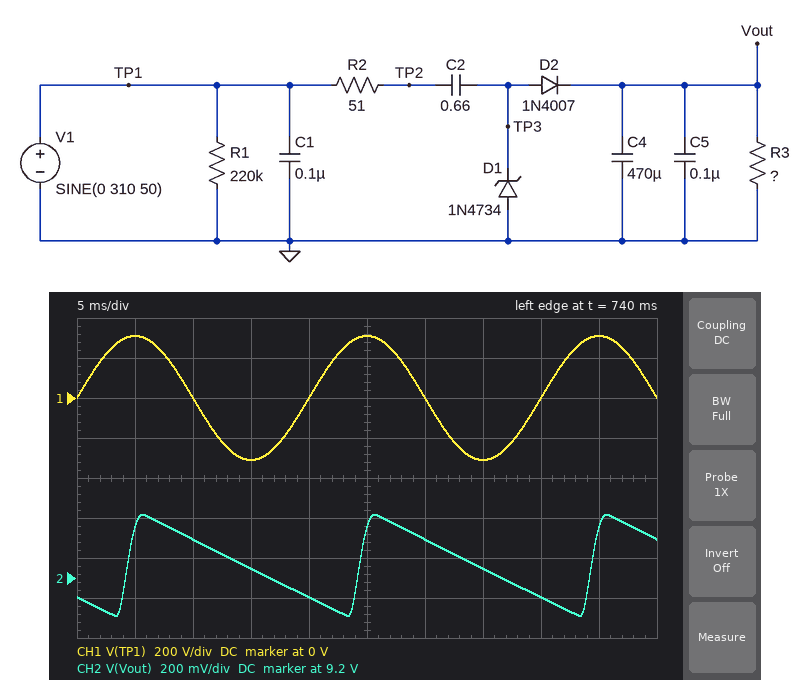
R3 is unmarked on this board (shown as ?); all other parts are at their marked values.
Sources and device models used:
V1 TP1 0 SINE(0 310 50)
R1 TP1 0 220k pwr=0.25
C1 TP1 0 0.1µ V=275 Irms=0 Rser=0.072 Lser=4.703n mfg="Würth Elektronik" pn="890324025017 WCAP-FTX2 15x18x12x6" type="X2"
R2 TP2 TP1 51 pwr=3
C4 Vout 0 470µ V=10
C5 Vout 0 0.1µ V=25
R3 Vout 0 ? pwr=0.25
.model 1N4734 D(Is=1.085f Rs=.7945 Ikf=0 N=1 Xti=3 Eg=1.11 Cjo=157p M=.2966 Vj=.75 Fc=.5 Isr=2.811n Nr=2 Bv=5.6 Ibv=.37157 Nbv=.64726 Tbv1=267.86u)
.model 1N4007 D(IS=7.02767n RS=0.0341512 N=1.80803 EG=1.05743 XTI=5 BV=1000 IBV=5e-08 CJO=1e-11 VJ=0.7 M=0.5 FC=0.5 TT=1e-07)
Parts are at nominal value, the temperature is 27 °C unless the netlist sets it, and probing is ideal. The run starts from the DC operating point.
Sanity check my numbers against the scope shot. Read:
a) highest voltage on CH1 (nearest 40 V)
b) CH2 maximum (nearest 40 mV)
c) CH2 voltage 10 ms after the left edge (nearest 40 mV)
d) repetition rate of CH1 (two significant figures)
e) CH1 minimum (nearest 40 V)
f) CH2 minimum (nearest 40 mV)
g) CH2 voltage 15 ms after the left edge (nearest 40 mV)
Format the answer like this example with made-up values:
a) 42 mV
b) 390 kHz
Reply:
a) 320 V
b) 9.52 V
c) 9.40 V
d) 50 Hz
e) -320 V
f) 9.00 V
g) 9.24 V
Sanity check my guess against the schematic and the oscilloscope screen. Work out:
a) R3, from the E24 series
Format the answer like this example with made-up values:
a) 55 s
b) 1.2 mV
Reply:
a) 680 Ω
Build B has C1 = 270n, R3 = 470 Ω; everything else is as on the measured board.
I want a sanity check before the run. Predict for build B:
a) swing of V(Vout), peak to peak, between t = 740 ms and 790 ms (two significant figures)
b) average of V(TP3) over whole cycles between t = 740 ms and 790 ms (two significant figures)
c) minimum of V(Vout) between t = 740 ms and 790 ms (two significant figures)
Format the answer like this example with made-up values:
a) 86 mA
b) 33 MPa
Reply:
a) 710 mV
b) 2.3 V
c) 8.8 V
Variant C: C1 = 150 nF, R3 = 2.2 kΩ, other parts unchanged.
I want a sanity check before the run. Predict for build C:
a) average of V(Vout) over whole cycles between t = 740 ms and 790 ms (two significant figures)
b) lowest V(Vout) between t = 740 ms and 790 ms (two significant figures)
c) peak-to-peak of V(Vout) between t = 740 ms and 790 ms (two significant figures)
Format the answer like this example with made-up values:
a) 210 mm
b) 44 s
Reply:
a) 9.5 V
b) 9.4 V
c) 160 mV
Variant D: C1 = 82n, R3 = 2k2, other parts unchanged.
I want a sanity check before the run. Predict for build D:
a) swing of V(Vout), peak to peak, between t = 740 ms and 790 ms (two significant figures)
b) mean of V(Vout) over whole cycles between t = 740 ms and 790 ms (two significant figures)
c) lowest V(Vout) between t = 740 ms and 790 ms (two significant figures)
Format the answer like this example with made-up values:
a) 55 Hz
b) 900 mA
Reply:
a) 160 mV
b) 9.5 V
c) 9.4 V
